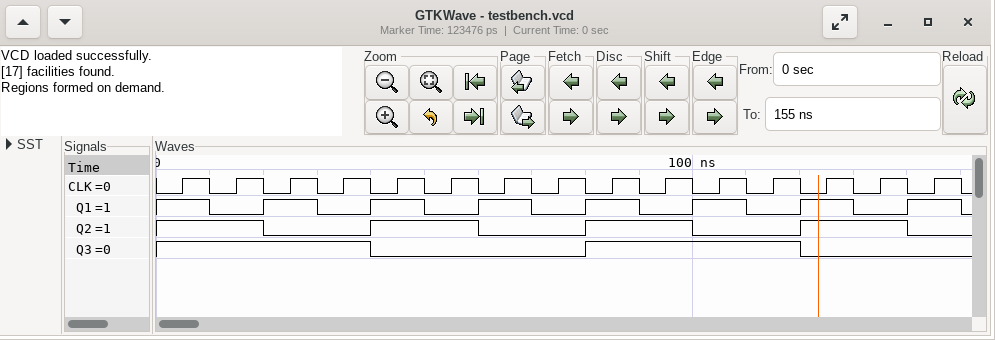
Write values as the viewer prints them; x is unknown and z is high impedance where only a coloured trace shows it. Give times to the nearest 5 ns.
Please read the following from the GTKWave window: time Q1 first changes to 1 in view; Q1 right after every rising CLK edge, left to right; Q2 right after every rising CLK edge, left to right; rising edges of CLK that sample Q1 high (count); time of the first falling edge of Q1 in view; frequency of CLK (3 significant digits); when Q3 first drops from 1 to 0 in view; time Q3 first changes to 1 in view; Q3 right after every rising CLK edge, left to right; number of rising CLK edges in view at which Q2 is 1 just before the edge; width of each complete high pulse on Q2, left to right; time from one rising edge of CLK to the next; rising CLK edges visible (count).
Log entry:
20 ns
1 0 1 0 1 0 1 0 1 0 1 0 1 0 1
1 1 0 0 1 1 0 0 1 1 0 0 1 1 0
8
10 ns
100 MHz
40 ns
80 ns
1 1 1 1 0 0 0 0 1 1 1 1 0 0 0
8
20 ns, 20 ns, 20 ns
10 ns
15
